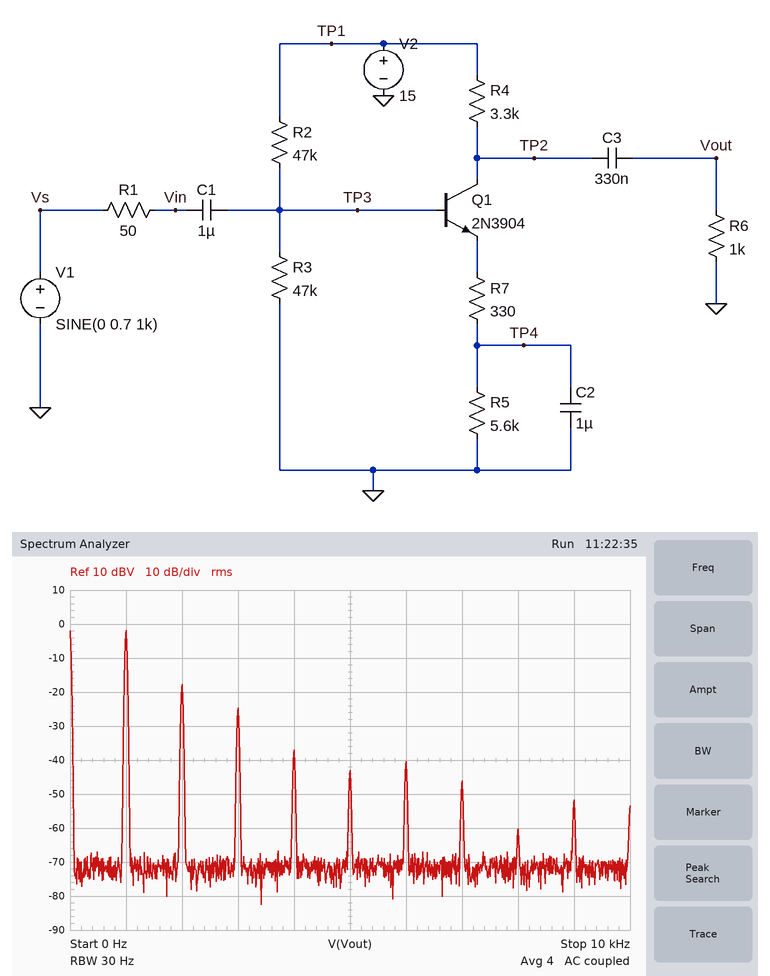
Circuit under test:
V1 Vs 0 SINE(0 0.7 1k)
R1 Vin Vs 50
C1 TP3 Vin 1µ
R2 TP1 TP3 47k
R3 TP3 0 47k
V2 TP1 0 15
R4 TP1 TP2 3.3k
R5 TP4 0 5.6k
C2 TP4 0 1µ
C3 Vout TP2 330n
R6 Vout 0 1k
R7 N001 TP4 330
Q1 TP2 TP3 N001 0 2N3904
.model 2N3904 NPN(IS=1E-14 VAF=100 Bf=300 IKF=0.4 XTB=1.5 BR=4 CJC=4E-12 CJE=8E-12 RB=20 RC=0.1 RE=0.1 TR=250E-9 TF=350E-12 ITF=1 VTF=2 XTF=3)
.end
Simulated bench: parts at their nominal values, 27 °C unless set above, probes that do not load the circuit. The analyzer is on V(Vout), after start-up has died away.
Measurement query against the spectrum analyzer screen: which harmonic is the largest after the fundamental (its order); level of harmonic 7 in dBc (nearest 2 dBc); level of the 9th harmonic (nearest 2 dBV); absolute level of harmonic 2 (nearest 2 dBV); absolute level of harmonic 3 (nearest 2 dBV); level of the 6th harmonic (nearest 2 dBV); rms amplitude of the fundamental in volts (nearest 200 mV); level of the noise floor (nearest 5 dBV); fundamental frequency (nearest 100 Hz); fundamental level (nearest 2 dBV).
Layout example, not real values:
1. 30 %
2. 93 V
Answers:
1. 2
2. -44 dBc
3. -52 dBV
4. -18 dBV
5. -24 dBV
6. -40 dBV
7. 800 mV
8. -70 dBV
9. 1.0 kHz
10. -2 dBV
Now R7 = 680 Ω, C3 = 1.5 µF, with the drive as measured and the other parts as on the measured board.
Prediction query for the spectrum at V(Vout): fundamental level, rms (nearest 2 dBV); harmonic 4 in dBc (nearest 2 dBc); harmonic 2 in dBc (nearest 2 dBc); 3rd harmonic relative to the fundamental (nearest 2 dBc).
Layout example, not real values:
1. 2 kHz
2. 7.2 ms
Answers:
1. -6 dBV
2. -54 dBc
3. -38 dBc
4. -46 dBc
